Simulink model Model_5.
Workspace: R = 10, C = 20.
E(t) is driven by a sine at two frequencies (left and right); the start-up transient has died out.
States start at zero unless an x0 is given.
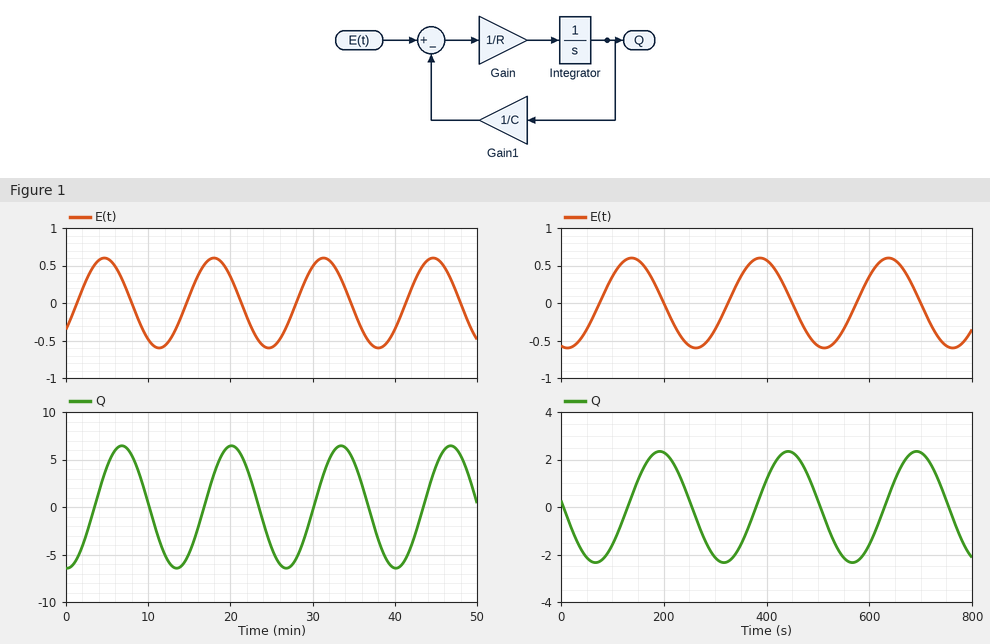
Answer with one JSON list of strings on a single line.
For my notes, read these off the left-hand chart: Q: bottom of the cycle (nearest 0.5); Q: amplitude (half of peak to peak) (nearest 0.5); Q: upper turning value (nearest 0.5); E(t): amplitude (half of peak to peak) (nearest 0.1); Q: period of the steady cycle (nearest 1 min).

["-6.5", "6.5", "6.5", "0.6", "13 min"]
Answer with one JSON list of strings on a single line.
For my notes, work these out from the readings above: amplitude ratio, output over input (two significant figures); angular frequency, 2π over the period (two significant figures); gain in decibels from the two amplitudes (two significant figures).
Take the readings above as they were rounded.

["11", "0.48 rad/min", "21 dB"]
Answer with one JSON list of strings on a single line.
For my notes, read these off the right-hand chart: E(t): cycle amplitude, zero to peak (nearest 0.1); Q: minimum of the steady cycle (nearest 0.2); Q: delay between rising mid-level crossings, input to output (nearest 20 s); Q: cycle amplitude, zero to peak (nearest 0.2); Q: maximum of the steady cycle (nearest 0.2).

["0.6", "-2.4", "60 s", "2.4", "2.4"]
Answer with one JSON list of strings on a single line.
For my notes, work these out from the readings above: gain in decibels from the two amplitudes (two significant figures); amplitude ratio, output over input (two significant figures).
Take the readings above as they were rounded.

["12 dB", "4.0"]
